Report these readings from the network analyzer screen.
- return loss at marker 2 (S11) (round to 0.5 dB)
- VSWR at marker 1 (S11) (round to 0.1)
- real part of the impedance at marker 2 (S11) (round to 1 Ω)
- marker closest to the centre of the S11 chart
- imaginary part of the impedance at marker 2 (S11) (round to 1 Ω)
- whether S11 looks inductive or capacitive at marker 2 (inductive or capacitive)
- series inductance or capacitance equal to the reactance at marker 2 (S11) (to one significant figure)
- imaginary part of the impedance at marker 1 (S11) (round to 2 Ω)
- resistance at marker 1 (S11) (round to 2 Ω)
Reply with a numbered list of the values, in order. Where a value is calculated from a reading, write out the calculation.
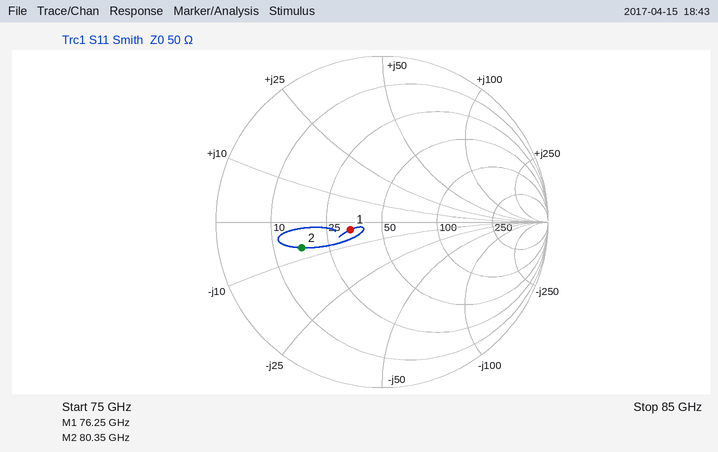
1. 6.0 dB
2. 1.5
3. 17 Ω
4. marker 1
5. -7 Ω
6. capacitive
7. C = 1/(2π × 80.35 GHz × 7 Ω) ≈ 283 fF, so 300 fF to one significant figure
8. -4 Ω
9. 34 Ω
